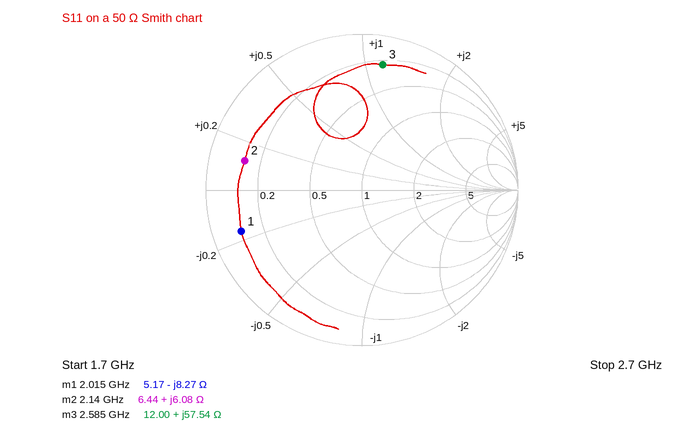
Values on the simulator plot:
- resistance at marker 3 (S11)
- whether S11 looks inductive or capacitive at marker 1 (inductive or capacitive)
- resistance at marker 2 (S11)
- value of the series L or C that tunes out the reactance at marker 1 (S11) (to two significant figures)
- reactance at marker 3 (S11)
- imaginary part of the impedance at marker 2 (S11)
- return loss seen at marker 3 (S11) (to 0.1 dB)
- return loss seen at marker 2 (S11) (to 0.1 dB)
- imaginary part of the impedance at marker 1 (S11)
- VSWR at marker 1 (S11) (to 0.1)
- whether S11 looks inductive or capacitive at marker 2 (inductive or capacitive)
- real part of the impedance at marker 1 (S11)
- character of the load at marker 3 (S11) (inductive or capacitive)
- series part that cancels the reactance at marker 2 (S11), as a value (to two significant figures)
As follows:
12.00 Ω
capacitive
6.44 Ω
650 pH
+57.54 Ω
+6.08 Ω
1.8 dB
2.2 dB
-8.27 Ω
9.9
inductive
5.17 Ω
inductive
12 pF
